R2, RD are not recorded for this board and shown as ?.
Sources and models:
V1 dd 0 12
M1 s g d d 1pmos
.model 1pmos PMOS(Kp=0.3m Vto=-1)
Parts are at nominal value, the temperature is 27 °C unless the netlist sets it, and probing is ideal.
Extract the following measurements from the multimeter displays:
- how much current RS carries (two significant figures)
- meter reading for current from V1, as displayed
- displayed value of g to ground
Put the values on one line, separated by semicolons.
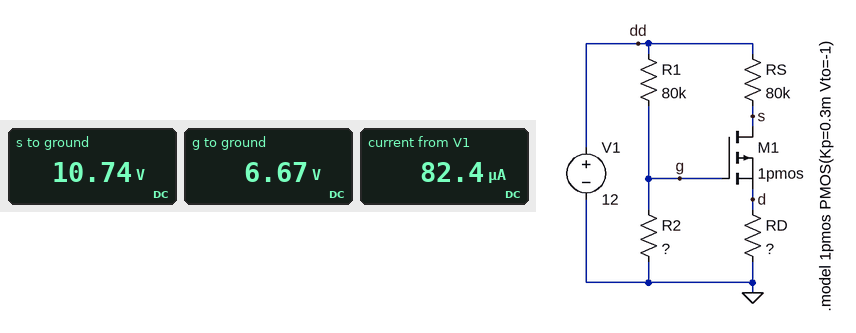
16 µA; 82.4 µA; 6.67 V
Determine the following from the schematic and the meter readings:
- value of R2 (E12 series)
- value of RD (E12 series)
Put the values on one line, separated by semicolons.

100 kΩ; 680 kΩ
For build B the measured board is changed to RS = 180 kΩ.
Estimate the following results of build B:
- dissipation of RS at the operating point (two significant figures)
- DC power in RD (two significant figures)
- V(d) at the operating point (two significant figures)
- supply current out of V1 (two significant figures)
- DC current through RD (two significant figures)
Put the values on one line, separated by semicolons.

35 µW; 130 µW; 9.5 V; 81 µA; 14 µA
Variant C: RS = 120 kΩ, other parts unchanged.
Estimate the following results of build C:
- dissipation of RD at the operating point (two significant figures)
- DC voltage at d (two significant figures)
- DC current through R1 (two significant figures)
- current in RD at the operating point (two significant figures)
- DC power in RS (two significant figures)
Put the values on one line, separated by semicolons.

150 µW; 10 V; 67 µA; 15 µA; 27 µW
